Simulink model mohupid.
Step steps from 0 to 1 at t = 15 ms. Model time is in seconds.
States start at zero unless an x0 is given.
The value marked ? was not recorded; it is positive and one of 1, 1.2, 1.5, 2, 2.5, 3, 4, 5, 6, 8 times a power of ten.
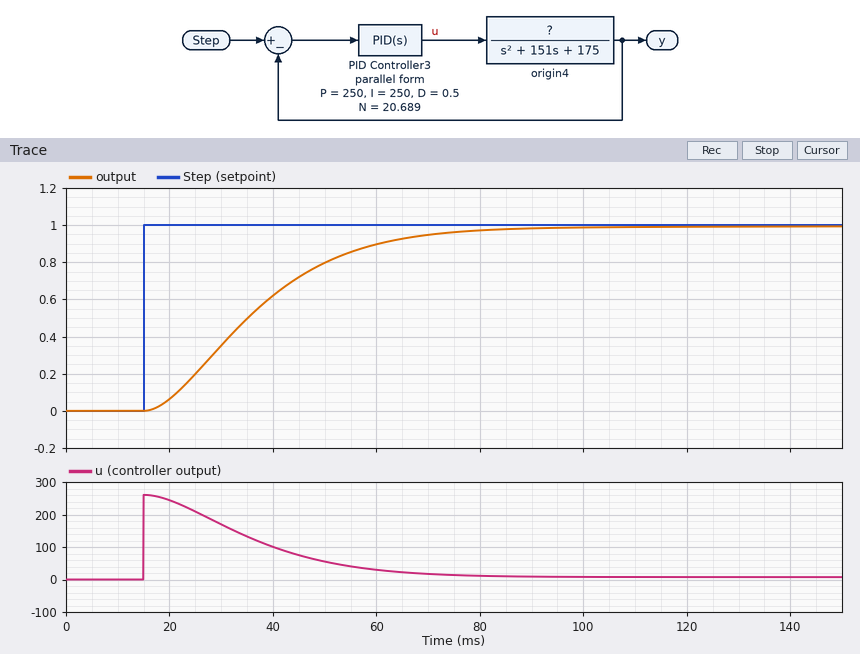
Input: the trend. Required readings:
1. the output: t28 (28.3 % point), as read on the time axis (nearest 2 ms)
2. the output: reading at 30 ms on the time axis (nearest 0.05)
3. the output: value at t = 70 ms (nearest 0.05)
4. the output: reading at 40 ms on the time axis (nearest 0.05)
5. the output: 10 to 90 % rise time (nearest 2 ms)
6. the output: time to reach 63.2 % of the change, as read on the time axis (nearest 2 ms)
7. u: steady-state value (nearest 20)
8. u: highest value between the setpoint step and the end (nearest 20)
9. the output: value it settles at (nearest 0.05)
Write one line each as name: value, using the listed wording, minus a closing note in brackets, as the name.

the output: t28 (28.3 % point), as read on the time axis: 28 ms
the output: reading at 30 ms on the time axis: 0.35
the output: value at t = 70 ms: 0.95
the output: reading at 40 ms on the time axis: 0.60
the output: 10 to 90 % rise time: 38 ms
the output: time to reach 63.2 % of the change, as read on the time axis: 40 ms
u: steady-state value: 0
u: highest value between the setpoint step and the end: 260
the output: value it settles at: 1.00
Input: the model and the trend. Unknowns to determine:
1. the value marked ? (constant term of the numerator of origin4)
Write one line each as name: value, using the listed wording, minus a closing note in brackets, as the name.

the value marked ?: 25
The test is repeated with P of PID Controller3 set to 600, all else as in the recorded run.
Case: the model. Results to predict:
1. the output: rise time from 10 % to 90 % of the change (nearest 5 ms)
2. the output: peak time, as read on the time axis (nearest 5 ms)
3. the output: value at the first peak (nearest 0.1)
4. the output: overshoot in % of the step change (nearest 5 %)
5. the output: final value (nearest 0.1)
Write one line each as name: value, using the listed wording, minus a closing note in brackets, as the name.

the output: rise time from 10 % to 90 % of the change: 15 ms
the output: peak time, as read on the time axis: 45 ms
the output: value at the first peak: 1.1
the output: overshoot in % of the step change: 10 %
the output: final value: 1.0
